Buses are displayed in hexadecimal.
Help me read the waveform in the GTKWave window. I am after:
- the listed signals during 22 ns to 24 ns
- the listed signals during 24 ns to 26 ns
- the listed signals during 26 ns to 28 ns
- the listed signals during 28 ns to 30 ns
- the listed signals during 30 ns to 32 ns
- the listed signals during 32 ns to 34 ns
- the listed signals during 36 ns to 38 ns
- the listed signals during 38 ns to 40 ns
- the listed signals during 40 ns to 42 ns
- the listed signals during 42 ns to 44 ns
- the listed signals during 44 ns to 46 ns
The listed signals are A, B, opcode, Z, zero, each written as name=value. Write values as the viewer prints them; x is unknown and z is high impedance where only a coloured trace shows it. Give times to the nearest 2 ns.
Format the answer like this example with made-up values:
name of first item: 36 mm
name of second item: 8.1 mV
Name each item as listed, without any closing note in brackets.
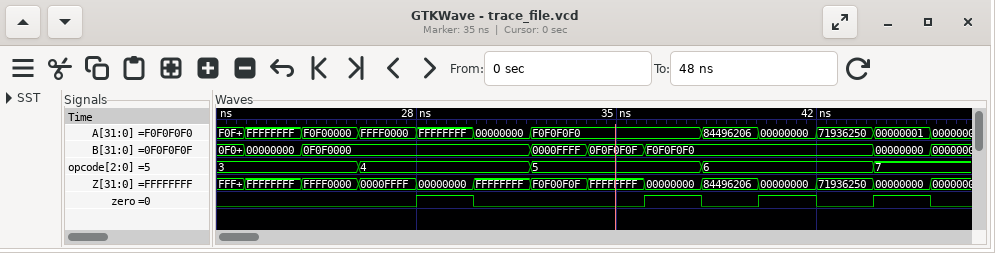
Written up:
the listed signals during 22 ns to 24 ns: A=FFFFFFFF, B=00000000, opcode=3, Z=FFFFFFFF, zero=0
the listed signals during 24 ns to 26 ns: A=F0F00000, B=0F0F0000, opcode=3, Z=FFFF0000, zero=0
the listed signals during 26 ns to 28 ns: A=FFFF0000, B=0F0F0000, opcode=4, Z=0000FFFF, zero=0
the listed signals during 28 ns to 30 ns: A=FFFFFFFF, B=0F0F0000, opcode=4, Z=00000000, zero=1
the listed signals during 30 ns to 32 ns: A=00000000, B=0F0F0000, opcode=4, Z=FFFFFFFF, zero=0
the listed signals during 32 ns to 34 ns: A=F0F0F0F0, B=0000FFFF, opcode=5, Z=F0F00F0F, zero=0
the listed signals during 36 ns to 38 ns: A=F0F0F0F0, B=F0F0F0F0, opcode=5, Z=00000000, zero=1
the listed signals during 38 ns to 40 ns: A=84496206, B=F0F0F0F0, opcode=6, Z=84496206, zero=0
the listed signals during 40 ns to 42 ns: A=00000000, B=F0F0F0F0, opcode=6, Z=00000000, zero=1
the listed signals during 42 ns to 44 ns: A=71936250, B=F0F0F0F0, opcode=6, Z=71936250, zero=0
the listed signals during 44 ns to 46 ns: A=00000001, B=00000000, opcode=7, Z=00000000, zero=1
